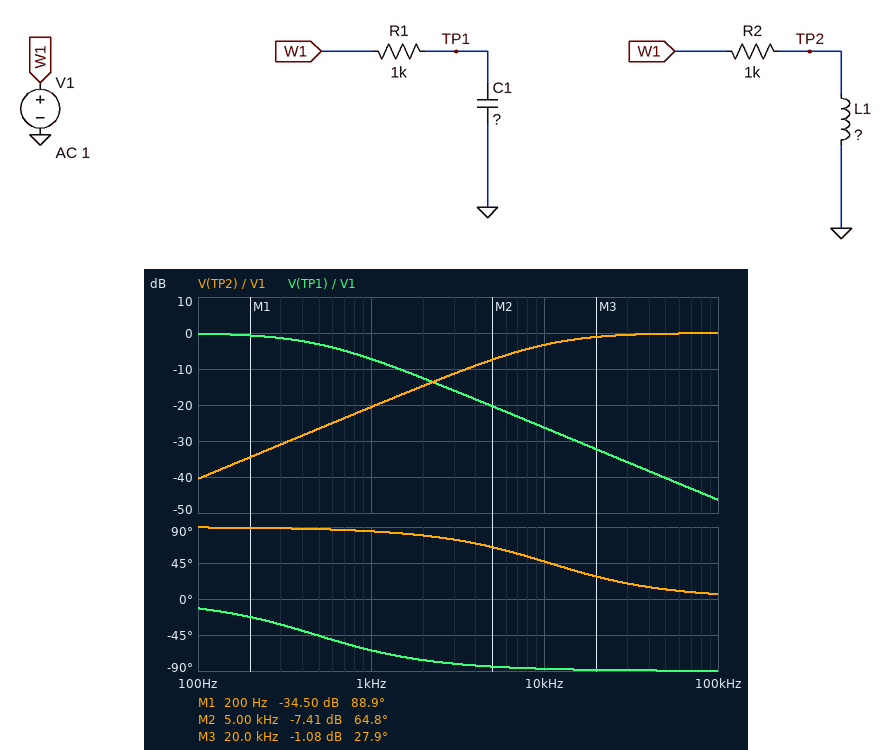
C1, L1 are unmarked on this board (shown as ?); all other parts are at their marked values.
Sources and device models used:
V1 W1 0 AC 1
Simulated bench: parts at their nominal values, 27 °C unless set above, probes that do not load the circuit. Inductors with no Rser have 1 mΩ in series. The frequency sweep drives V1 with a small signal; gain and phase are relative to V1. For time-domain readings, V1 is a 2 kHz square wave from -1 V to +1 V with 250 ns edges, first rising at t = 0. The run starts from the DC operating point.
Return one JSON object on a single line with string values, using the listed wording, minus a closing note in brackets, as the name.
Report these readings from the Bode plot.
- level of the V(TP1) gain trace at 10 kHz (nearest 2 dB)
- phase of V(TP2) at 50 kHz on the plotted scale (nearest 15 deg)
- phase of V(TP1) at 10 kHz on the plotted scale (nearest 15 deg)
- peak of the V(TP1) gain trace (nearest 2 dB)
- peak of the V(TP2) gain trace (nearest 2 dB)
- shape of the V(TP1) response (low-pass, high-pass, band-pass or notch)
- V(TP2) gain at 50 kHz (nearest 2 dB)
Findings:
{"level of the V(TP1) gain trace at 10 kHz": "-26 dB", "phase of V(TP2) at 50 kHz on the plotted scale": "15 deg", "phase of V(TP1) at 10 kHz on the plotted scale": "-90 deg", "peak of the V(TP1) gain trace": "0 dB", "peak of the V(TP2) gain trace": "0 dB", "shape of the V(TP1) response": "low-pass", "V(TP2) gain at 50 kHz": "0 dB"}
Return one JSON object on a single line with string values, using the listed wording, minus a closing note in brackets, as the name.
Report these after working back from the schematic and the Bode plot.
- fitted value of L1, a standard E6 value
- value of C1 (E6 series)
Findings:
{"fitted value of L1, a standard E6 value": "15 mH", "value of C1": "330 nF"}
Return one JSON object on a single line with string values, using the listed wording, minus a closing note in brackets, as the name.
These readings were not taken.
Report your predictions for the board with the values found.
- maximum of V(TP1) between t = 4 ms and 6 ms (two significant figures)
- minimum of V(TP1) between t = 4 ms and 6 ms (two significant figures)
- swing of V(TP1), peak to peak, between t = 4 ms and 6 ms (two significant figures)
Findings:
{"maximum of V(TP1) between t = 4 ms and 6 ms": "360 mV", "minimum of V(TP1) between t = 4 ms and 6 ms": "-360 mV", "swing of V(TP1), peak to peak, between t = 4 ms and 6 ms": "720 mV"}
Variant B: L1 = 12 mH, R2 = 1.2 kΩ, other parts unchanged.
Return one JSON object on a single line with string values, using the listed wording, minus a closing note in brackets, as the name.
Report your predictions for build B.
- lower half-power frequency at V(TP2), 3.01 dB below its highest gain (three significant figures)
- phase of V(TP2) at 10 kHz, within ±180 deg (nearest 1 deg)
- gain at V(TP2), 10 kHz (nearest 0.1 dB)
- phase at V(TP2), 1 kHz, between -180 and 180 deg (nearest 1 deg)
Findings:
{"lower half-power frequency at V(TP2), 3.01 dB below its highest gain": "15.9 kHz", "phase of V(TP2) at 10 kHz, within ±180 deg": "58 deg", "gain at V(TP2), 10 kHz": "-5.5 dB", "phase at V(TP2), 1 kHz, between -180 and 180 deg": "86 deg"}
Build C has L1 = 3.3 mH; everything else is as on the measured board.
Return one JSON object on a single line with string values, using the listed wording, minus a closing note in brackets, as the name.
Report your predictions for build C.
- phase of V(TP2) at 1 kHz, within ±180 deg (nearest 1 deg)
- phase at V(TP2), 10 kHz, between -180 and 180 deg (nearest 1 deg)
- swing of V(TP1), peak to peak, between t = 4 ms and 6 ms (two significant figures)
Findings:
{"phase of V(TP2) at 1 kHz, within ±180 deg": "89 deg", "phase at V(TP2), 10 kHz, between -180 and 180 deg": "78 deg", "swing of V(TP1), peak to peak, between t = 4 ms and 6 ms": "720 mV"}
